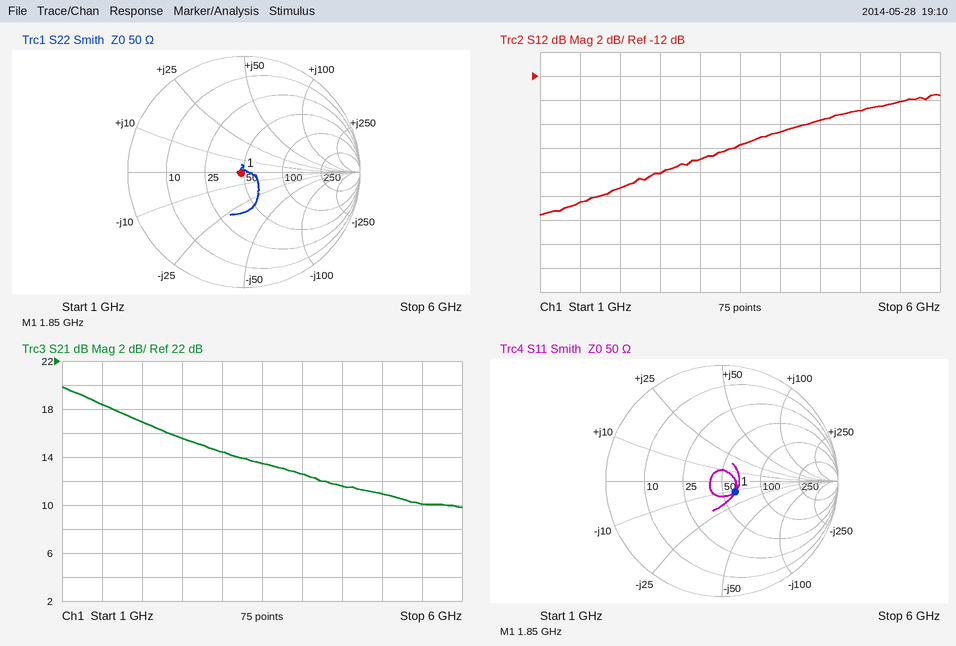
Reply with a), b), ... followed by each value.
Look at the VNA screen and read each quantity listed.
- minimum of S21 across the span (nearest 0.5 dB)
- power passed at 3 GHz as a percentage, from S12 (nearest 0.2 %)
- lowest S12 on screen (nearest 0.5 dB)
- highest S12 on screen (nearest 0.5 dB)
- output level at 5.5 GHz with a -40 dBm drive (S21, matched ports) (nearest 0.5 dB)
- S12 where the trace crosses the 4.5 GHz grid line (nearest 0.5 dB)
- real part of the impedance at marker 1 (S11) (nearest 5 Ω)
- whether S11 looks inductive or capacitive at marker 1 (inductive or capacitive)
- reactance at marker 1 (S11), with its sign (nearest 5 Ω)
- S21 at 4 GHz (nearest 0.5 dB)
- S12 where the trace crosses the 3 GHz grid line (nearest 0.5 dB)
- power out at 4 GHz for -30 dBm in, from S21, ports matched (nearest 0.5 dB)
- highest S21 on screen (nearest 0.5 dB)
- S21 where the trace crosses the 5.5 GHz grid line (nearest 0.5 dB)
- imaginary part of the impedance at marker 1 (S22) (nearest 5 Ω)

a) 10.0 dB
b) 1.2 %
c) -23.5 dB
d) -13.5 dB
e) -30.0 dBm
f) -15.5 dB
g) 60 Ω
h) capacitive
i) -10 Ω
j) 12.5 dB
k) -19.0 dB
l) -17.5 dBm
m) 20.0 dB
n) 10.0 dB
o) 0 Ω
